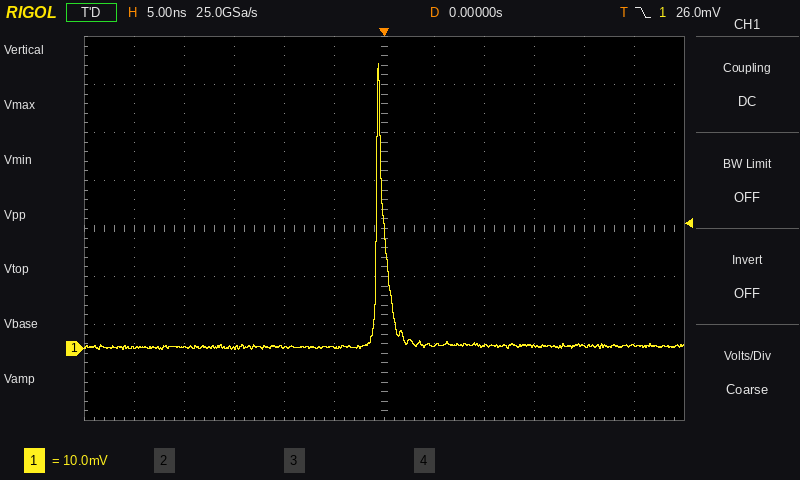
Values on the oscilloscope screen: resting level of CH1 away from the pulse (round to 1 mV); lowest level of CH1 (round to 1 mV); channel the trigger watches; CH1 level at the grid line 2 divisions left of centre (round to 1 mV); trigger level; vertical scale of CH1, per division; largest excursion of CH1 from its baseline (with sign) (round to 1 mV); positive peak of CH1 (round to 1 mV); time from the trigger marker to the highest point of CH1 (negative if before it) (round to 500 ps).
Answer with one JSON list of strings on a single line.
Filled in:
["0 mV", "0 mV", "CH1", "0 mV", "26.0 mV", "10 mV", "+59 mV", "59 mV", "-500 ps"]
